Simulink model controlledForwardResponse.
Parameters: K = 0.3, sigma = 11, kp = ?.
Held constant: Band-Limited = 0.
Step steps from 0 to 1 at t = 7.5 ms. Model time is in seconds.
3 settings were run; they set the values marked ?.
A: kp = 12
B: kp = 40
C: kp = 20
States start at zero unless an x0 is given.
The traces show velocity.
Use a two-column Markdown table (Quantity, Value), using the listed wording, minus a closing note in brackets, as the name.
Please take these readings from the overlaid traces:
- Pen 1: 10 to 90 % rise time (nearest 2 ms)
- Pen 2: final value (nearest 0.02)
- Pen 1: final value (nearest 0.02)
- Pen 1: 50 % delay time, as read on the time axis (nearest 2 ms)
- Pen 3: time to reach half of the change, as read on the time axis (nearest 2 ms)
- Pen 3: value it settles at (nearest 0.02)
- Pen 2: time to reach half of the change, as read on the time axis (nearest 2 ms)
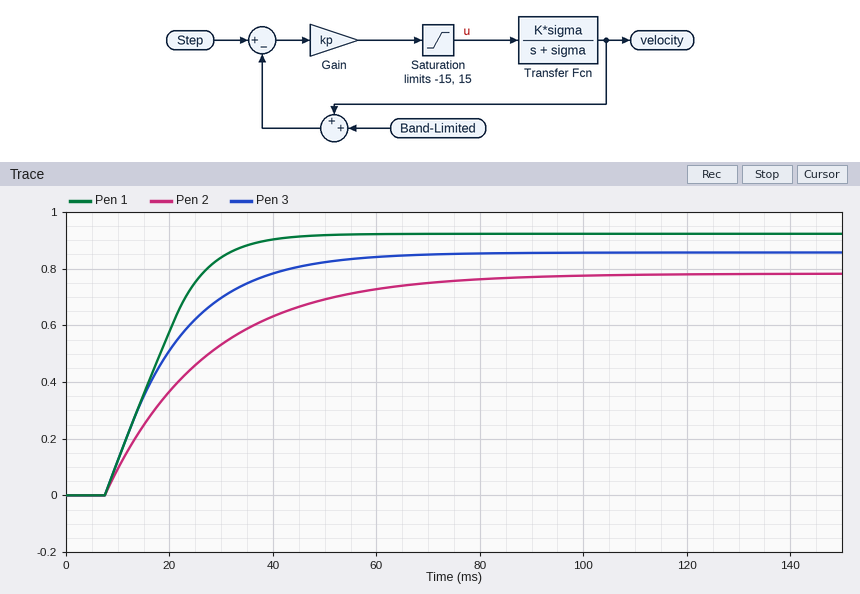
| Quantity | Value |
|---|---|
| Pen 1: 10 to 90 % rise time | 20 ms |
| Pen 2: final value | 0.78 |
| Pen 1: final value | 0.92 |
| Pen 1: 50 % delay time, as read on the time axis | 18 ms |
| Pen 3: time to reach half of the change, as read on the time axis | 18 ms |
| Pen 3: value it settles at | 0.86 |
| Pen 2: time to reach half of the change, as read on the time axis | 22 ms |
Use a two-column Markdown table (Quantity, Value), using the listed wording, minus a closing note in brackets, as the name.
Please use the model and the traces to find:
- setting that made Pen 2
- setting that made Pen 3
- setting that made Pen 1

| Quantity | Value |
|---|---|
| setting that made Pen 2 | A |
| setting that made Pen 3 | C |
| setting that made Pen 1 | B |
